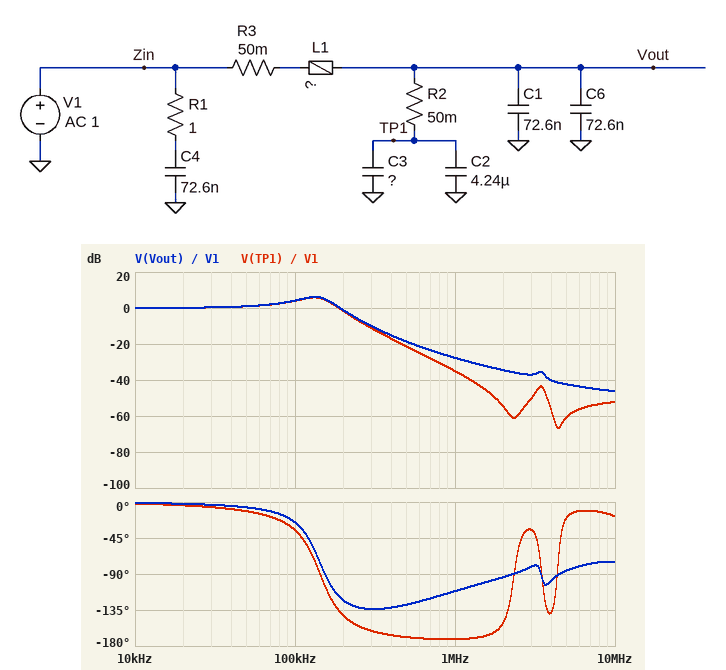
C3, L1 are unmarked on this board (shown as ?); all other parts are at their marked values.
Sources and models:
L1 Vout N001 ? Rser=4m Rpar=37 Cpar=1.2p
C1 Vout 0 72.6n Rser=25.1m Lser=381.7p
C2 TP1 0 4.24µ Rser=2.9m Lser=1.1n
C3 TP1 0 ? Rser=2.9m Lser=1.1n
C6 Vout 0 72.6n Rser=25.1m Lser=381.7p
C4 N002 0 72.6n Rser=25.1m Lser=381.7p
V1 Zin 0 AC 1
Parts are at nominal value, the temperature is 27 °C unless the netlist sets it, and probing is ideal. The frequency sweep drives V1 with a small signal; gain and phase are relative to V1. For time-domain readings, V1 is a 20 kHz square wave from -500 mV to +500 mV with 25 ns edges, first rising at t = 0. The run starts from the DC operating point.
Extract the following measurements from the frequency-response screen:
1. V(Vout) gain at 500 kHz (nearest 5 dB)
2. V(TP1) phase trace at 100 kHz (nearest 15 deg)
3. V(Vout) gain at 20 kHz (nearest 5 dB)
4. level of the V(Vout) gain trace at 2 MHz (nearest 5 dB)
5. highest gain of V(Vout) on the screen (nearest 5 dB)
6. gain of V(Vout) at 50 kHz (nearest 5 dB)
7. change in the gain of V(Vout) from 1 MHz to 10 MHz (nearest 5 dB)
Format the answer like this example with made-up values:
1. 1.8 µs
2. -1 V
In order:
1. -20 dB
2. -30 deg
3. 0 dB
4. -35 dB
5. 5 dB
6. 0 dB
7. -20 dB
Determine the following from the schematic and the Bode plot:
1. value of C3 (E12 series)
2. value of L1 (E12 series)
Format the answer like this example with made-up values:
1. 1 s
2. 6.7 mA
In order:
1. 1.2 µF
2. 220 nH
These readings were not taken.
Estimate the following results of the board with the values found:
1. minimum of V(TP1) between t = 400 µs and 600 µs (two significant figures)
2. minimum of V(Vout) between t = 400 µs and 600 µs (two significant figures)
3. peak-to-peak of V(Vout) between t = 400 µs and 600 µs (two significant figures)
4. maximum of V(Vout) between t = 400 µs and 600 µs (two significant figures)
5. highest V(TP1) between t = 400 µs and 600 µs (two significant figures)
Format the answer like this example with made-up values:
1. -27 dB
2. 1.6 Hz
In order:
1. -930 mV
2. -940 mV
3. 1.9 V
4. 940 mV
5. 930 mV
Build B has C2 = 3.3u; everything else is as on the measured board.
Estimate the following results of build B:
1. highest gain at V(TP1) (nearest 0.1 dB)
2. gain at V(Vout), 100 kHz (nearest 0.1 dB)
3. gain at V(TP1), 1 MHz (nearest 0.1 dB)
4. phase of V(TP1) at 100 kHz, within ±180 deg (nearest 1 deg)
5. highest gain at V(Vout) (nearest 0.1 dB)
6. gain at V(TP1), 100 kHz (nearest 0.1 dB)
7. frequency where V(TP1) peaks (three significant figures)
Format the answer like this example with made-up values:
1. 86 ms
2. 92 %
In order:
1. 6.7 dB
2. 3.6 dB
3. -33.0 dB
4. -27 deg
5. 6.9 dB
6. 3.5 dB
7. 148 kHz
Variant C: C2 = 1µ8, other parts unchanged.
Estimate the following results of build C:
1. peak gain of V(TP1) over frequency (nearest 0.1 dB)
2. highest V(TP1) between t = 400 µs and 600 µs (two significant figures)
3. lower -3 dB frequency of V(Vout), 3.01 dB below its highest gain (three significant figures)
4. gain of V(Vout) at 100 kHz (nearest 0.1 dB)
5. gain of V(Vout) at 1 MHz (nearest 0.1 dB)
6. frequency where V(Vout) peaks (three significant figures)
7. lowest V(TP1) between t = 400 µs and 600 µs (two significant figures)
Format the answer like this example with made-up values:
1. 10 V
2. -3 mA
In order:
1. 8.4 dB
2. 1.0 V
3. 141 kHz
4. 2.5 dB
5. -25.9 dB
6. 184 kHz
7. -1.0 V
